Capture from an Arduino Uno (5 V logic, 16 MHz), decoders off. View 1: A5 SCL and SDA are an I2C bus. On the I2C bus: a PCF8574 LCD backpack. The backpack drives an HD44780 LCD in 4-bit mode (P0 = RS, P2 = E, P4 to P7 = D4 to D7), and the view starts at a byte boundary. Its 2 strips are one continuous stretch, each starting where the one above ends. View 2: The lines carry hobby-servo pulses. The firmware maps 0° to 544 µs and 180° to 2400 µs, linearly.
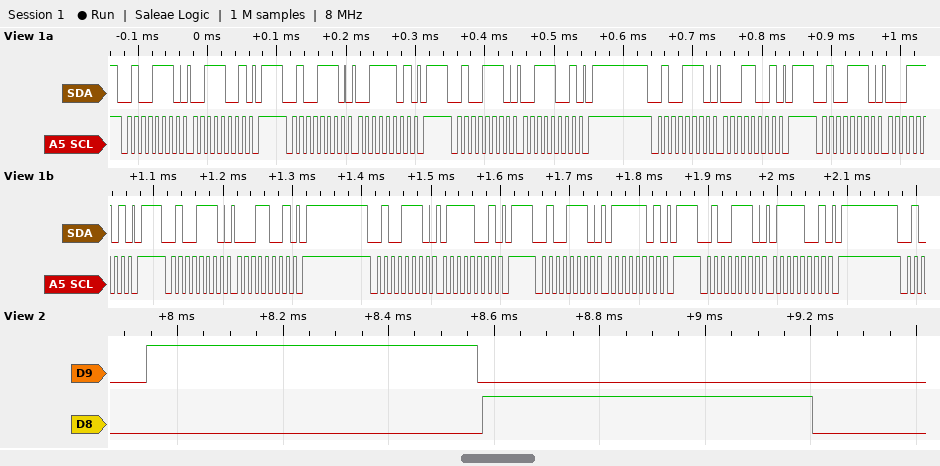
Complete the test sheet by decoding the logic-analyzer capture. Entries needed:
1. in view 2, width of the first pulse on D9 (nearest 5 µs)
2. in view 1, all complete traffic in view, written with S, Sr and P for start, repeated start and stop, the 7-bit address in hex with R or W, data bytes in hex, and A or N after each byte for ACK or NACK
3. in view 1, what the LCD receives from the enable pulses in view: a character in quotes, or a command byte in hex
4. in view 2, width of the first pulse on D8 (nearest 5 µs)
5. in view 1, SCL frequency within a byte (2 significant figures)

625 µs
S 27W A 39 A P S 27W A 3D A P S 27W A 39 A P S 27W A 19 A P S 27W A 1D A P S 27W A 19 A P S 27W A 79 A P S 27W A 7D A P S 27W A 79 A P
'1'
625 µs
100 kHz
